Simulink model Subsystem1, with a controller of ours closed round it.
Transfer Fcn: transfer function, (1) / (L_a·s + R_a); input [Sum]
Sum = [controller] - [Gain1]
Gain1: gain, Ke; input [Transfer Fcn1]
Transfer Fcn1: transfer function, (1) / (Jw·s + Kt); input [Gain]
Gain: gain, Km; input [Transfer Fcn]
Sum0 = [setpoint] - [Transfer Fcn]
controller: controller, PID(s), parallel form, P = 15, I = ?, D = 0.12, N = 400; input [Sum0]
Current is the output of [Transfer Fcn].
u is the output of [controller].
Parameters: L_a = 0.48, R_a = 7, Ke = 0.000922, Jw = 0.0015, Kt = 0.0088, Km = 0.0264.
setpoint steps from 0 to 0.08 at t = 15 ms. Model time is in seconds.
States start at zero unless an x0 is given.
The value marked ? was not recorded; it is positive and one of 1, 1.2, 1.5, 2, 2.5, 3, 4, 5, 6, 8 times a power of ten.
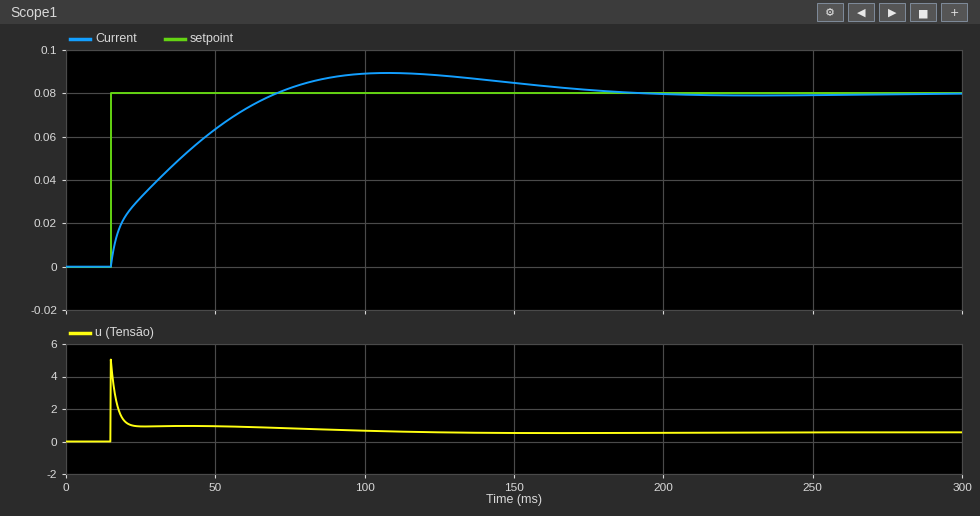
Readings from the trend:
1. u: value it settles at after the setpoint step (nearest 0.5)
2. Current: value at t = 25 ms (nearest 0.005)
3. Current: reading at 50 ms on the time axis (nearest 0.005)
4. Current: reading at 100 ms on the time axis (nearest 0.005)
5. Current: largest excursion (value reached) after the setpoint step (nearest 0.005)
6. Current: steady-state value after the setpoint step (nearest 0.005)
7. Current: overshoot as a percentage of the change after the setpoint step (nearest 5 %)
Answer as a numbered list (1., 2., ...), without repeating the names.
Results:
1. 0.5
2. 0.030
3. 0.065
4. 0.090
5. 0.090
6. 0.080
7. 10 %
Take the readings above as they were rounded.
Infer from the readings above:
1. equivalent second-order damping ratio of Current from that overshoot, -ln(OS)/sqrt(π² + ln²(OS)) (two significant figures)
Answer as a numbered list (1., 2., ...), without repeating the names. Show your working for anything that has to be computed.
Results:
1. ln(0.1) = -2.303; 2.303 / sqrt(9.870 + 5.302) = 0.59
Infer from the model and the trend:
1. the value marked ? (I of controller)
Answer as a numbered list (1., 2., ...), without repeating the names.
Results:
1. 600
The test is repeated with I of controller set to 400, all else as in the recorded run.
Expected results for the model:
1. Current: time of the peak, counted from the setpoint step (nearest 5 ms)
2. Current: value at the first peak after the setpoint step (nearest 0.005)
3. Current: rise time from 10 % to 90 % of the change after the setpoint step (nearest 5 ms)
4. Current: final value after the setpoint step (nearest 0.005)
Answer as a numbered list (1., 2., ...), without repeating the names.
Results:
1. 120 ms
2. 0.085
3. 55 ms
4. 0.080
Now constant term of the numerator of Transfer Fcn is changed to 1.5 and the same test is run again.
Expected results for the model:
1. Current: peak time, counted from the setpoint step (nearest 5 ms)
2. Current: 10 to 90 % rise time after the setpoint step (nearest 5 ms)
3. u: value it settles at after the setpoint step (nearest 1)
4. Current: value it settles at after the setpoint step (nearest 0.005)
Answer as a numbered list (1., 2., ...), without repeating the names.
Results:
1. 75 ms
2. 35 ms
3. 0
4. 0.080
